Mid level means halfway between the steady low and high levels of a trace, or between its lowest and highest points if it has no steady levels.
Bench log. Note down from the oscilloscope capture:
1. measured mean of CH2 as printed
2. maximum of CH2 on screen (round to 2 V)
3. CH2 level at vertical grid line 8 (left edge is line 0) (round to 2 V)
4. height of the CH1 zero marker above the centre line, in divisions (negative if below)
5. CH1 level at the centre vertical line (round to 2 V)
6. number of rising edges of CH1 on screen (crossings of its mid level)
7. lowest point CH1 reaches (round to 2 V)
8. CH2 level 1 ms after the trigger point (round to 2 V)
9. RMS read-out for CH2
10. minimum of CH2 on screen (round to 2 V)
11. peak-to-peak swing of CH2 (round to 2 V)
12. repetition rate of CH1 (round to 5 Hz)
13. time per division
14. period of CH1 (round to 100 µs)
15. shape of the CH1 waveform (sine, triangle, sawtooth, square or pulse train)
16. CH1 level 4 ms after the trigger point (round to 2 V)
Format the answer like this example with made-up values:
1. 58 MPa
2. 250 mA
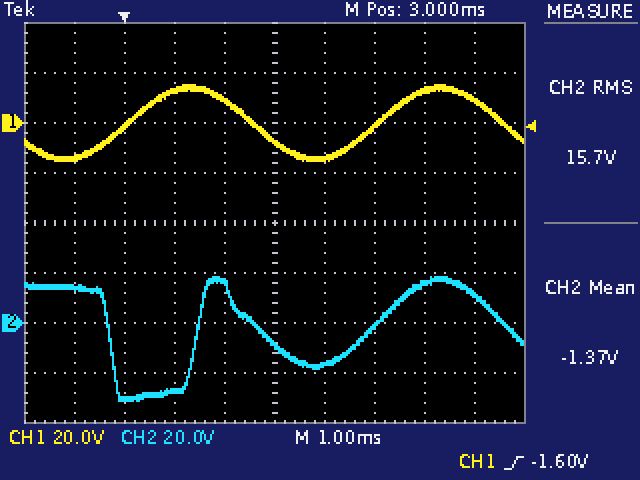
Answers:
1. -1.37 V
2. 18 V
3. 16 V
4. +2.0 div
5. -8 V
6. 2
7. -16 V
8. -28 V
9. 15.7 V
10. -32 V
11. 50 V
12. 200 Hz
13. 1 ms
14. 5.0 ms
15. sine
16. -14 V
